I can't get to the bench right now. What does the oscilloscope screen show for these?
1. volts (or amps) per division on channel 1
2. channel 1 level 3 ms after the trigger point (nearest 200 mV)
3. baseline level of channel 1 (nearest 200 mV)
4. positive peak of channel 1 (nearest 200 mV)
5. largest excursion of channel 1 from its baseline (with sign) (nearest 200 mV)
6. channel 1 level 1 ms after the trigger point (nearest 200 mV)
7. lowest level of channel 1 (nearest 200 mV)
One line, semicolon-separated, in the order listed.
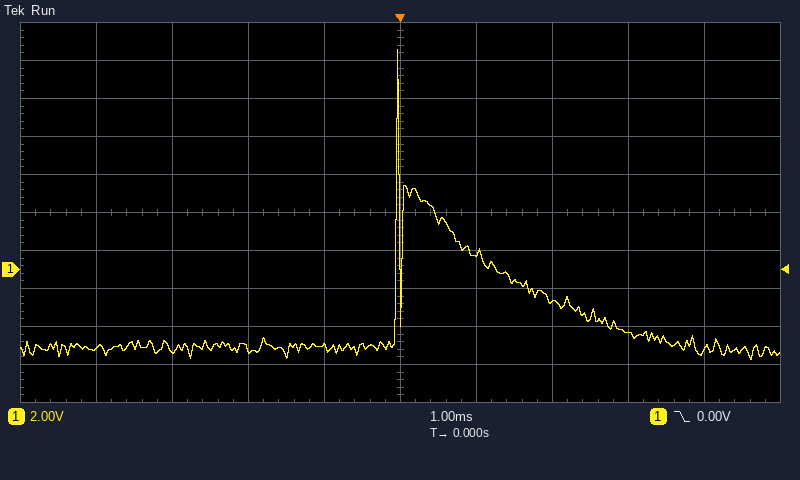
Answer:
2 V; -3.4 V; -4.0 V; 11.6 V; +15.6 V; 800 mV; -4.8 V
